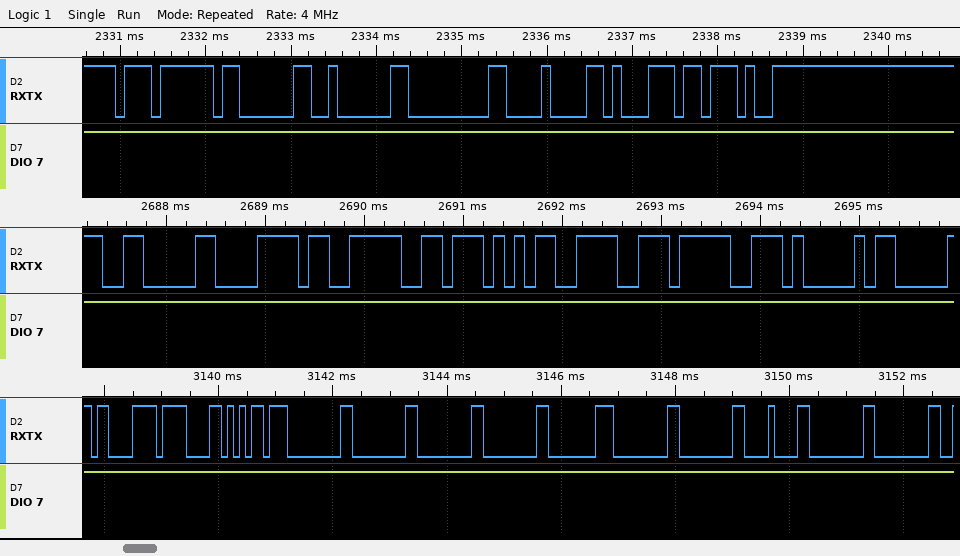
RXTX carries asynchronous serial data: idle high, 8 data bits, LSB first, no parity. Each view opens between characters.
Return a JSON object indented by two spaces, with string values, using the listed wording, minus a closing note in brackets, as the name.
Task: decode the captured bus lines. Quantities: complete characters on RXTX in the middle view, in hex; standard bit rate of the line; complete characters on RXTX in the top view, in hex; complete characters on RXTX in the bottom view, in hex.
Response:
{
  "complete characters on RXTX in the middle view, in hex": "06, 78, 3E, 57, 9E, 9F, 41",
  "standard bit rate of the line": "9600 baud",
  "complete characters on RXTX in the top view, in hex": "F7, 03, 02, 00, 08, 71, 97",
  "complete characters on RXTX in the bottom view, in hex": "C3, 0F, B5, 00, 00, 00, 00, 80, 00, 00, 08, 00, 00"
}
